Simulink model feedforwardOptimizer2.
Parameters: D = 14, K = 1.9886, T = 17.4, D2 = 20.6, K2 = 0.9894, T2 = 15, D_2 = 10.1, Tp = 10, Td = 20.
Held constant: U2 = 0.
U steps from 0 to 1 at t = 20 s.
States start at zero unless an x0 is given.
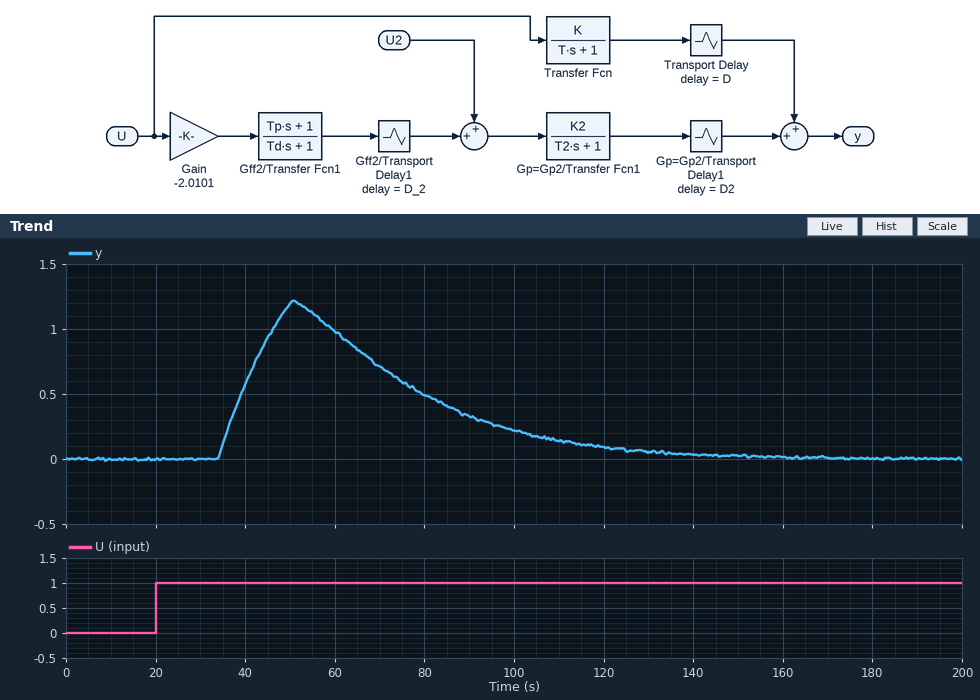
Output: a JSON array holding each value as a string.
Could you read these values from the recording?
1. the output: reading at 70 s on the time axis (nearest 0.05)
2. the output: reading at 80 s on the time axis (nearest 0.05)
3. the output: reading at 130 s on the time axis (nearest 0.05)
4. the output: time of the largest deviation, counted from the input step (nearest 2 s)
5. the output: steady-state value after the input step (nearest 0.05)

["0.70", "0.50", "0.05", "30 s", "0.00"]
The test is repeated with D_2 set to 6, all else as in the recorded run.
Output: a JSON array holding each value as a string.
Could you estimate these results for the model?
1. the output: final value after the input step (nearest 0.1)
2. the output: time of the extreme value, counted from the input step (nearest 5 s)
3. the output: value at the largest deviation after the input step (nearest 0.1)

["0.0", "25 s", "1.0"]
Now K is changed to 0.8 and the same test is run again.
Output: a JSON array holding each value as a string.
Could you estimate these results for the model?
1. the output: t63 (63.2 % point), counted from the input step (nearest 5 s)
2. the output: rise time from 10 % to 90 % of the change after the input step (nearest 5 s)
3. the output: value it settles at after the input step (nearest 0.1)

["65 s", "50 s", "-1.2"]
